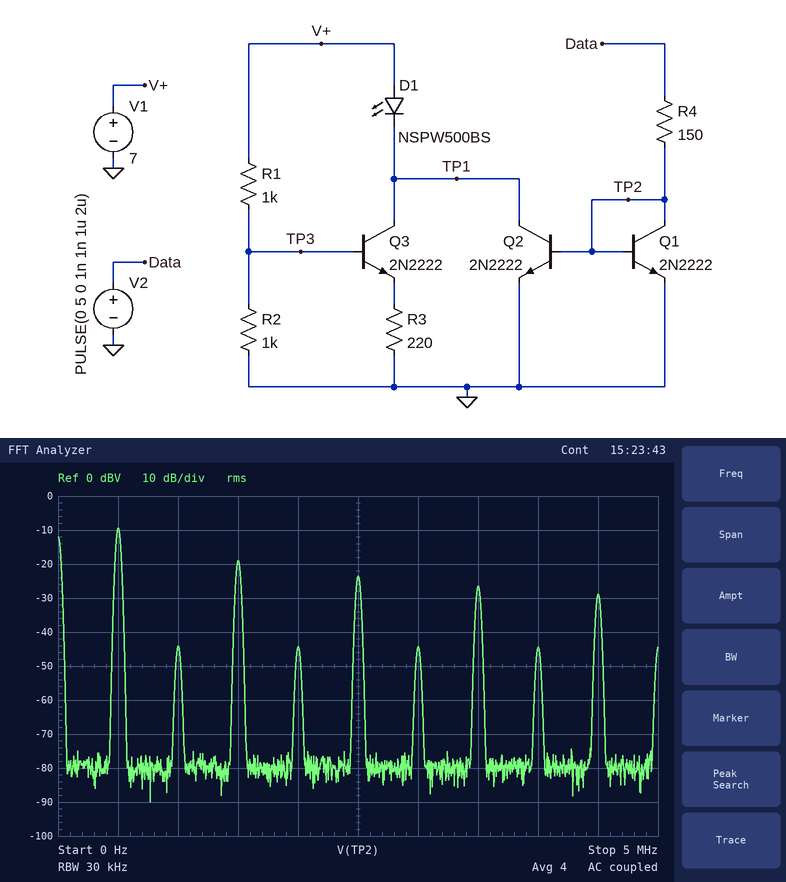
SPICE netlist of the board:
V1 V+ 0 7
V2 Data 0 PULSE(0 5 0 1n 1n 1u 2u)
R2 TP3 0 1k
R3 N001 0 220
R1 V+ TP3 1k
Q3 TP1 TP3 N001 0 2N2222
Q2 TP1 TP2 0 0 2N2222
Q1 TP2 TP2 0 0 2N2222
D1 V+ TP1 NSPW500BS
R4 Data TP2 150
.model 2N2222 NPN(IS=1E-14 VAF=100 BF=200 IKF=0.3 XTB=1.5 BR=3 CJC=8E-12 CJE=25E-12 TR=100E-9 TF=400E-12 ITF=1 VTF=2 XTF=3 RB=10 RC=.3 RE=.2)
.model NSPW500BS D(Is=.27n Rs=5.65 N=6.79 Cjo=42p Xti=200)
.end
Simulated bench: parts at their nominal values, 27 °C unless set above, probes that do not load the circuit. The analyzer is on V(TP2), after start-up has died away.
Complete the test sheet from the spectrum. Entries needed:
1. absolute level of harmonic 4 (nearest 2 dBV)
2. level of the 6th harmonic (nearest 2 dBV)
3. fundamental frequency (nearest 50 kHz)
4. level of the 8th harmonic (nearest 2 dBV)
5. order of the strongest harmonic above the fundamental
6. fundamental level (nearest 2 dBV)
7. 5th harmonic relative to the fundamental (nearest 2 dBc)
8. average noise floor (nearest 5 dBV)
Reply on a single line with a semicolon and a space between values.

-44 dBV; -44 dBV; 500 kHz; -44 dBV; 3; -10 dBV; -14 dBc; -80 dBV
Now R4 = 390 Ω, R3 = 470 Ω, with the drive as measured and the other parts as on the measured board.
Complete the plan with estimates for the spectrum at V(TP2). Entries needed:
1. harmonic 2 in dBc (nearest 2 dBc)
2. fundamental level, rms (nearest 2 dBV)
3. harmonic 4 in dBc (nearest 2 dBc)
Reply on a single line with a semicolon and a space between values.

-28 dBc; -10 dBV; -28 dBc
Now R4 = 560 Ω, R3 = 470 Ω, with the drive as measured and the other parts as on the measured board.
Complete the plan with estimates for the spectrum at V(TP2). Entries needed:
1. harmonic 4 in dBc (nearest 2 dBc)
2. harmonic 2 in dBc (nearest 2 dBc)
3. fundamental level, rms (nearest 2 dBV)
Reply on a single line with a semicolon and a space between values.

-26 dBc; -26 dBc; -10 dBV
